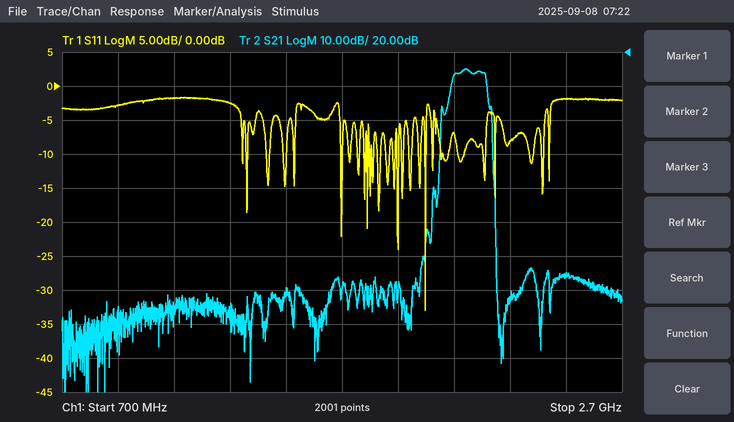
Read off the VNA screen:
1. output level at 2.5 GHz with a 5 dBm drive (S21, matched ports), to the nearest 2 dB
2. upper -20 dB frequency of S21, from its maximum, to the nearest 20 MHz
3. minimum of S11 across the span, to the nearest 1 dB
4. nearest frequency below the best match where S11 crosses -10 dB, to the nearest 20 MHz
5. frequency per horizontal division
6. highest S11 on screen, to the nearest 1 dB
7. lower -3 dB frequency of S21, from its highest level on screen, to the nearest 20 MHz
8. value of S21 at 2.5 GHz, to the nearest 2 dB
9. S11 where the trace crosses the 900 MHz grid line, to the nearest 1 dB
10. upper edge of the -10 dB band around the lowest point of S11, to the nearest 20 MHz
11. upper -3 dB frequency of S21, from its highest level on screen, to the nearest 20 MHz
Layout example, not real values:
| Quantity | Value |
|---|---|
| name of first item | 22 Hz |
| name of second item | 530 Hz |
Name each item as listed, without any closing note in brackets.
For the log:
| Quantity | Value |
|---|---|
| output level at 2.5 GHz with a 5 dBm drive (S21, matched ports), to the nearest 2 dB | -40 dBm |
| upper -20 dB frequency of S21, from its maximum, to the nearest 20 MHz | 2.24 GHz |
| minimum of S11 across the span, to the nearest 1 dB | -33 dB |
| nearest frequency below the best match where S11 crosses -10 dB, to the nearest 20 MHz | 2.00 GHz |
| frequency per horizontal division | 200 MHz |
| highest S11 on screen, to the nearest 1 dB | -2 dB |
| lower -3 dB frequency of S21, from its highest level on screen, to the nearest 20 MHz | 2.10 GHz |
| value of S21 at 2.5 GHz, to the nearest 2 dB | -46 dB |
| S11 where the trace crosses the 900 MHz grid line, to the nearest 1 dB | -3 dB |
| upper edge of the -10 dB band around the lowest point of S11, to the nearest 20 MHz | 2.00 GHz |
| upper -3 dB frequency of S21, from its highest level on screen, to the nearest 20 MHz | 2.22 GHz |
